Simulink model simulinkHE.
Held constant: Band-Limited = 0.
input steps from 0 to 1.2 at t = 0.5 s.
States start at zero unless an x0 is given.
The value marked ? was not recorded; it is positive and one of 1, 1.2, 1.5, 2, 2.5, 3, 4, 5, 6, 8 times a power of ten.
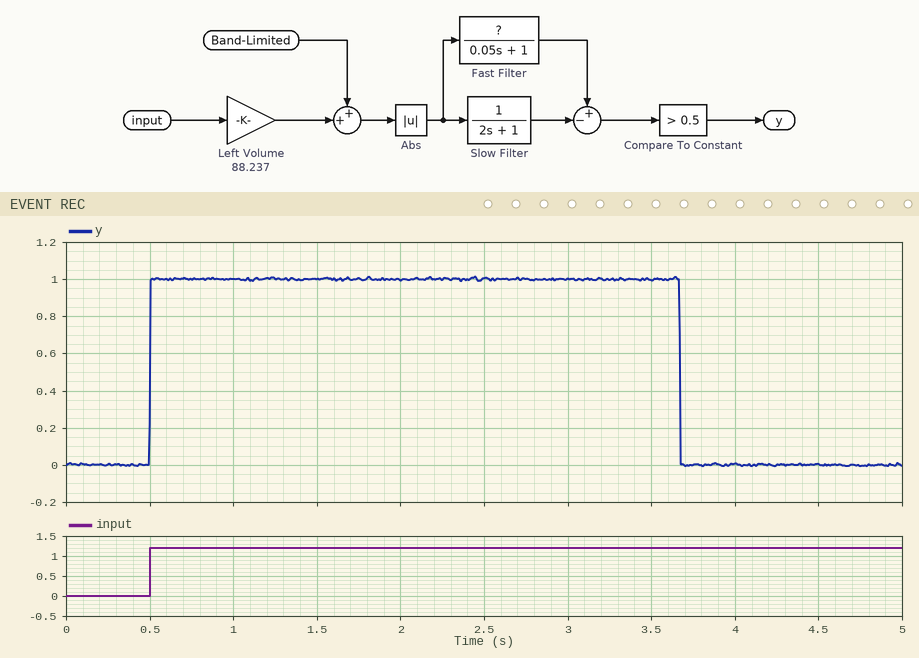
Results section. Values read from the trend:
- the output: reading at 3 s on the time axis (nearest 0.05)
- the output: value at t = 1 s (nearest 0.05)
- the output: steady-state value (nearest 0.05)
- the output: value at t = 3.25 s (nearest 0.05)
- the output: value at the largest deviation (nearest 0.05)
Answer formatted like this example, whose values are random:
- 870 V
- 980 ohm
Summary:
- 1.00
- 1.00
- 0.00
- 1.00
- 1.00
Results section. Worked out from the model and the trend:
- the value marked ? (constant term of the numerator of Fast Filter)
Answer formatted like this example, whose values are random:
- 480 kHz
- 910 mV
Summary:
- 0.8
